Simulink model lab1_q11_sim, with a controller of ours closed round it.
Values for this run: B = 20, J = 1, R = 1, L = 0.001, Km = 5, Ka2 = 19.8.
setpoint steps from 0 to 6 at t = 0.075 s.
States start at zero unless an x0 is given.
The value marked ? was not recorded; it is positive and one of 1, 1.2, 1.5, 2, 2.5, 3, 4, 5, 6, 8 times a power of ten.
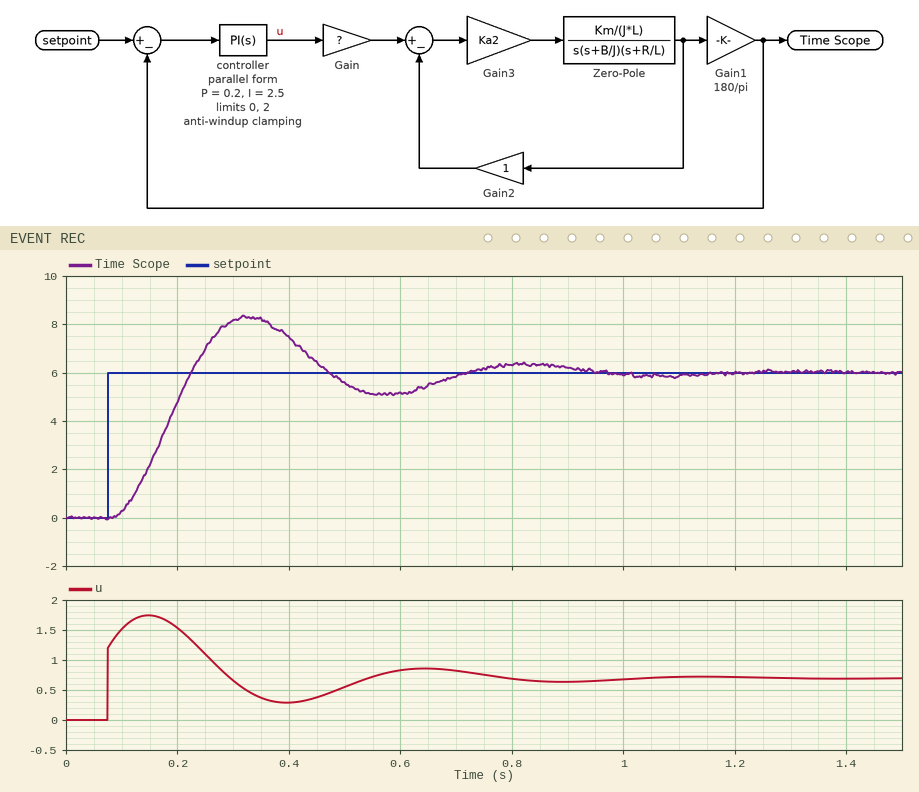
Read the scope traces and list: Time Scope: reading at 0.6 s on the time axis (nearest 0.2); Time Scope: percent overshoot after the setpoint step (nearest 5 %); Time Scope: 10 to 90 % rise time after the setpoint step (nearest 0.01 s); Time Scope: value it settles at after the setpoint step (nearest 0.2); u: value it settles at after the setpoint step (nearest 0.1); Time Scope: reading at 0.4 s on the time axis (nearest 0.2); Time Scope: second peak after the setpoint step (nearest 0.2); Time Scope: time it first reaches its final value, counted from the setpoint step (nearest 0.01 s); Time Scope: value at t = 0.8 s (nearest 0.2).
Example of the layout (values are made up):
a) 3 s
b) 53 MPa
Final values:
a) 5.2
b) 40 %
c) 0.10 s
d) 6.0
e) 0.7
f) 7.4
g) 6.4
h) 0.15 s
i) 6.4
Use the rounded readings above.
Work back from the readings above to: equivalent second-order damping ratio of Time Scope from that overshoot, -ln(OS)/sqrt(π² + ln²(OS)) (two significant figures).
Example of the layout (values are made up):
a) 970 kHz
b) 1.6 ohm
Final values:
a) 0.28
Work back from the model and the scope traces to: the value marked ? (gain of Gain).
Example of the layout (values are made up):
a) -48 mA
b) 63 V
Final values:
a) 0.15
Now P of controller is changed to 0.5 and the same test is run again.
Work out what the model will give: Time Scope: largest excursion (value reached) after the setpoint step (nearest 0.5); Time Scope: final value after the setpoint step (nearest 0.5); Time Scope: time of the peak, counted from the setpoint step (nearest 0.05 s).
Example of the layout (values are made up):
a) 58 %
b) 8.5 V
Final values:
a) 6.5
b) 6.0
c) 0.20 s
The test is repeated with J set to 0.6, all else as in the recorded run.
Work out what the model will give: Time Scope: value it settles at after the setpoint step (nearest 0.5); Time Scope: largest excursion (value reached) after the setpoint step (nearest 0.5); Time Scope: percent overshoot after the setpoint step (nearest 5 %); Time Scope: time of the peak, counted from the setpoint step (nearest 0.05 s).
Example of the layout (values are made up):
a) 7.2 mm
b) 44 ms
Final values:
a) 6.0
b) 7.5
c) 25 %
d) 0.25 s
